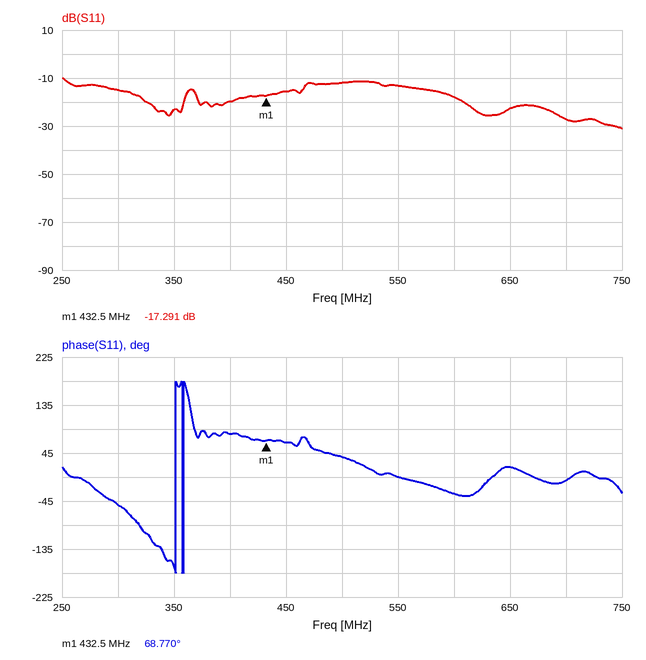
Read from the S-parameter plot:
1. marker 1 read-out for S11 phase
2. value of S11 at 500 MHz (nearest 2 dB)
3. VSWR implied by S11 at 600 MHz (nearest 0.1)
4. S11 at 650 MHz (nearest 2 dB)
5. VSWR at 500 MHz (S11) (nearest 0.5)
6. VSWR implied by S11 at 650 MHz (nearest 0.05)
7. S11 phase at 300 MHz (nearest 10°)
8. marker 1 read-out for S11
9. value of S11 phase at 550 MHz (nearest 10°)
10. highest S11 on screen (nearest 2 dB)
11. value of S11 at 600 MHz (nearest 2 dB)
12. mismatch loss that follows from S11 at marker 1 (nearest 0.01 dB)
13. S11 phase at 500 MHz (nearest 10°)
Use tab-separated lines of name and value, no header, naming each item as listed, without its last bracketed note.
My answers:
marker 1 read-out for S11 phase	68.770°
value of S11 at 500 MHz	-12 dB
VSWR implied by S11 at 600 MHz	1.3
S11 at 650 MHz	-22 dB
VSWR at 500 MHz (S11)	1.5
VSWR implied by S11 at 650 MHz	1.15
S11 phase at 300 MHz	-50°
marker 1 read-out for S11	-17.291 dB
value of S11 phase at 550 MHz	0°
highest S11 on screen	-10 dB
value of S11 at 600 MHz	-18 dB
mismatch loss that follows from S11 at marker 1	0.08 dB
S11 phase at 500 MHz	40°
